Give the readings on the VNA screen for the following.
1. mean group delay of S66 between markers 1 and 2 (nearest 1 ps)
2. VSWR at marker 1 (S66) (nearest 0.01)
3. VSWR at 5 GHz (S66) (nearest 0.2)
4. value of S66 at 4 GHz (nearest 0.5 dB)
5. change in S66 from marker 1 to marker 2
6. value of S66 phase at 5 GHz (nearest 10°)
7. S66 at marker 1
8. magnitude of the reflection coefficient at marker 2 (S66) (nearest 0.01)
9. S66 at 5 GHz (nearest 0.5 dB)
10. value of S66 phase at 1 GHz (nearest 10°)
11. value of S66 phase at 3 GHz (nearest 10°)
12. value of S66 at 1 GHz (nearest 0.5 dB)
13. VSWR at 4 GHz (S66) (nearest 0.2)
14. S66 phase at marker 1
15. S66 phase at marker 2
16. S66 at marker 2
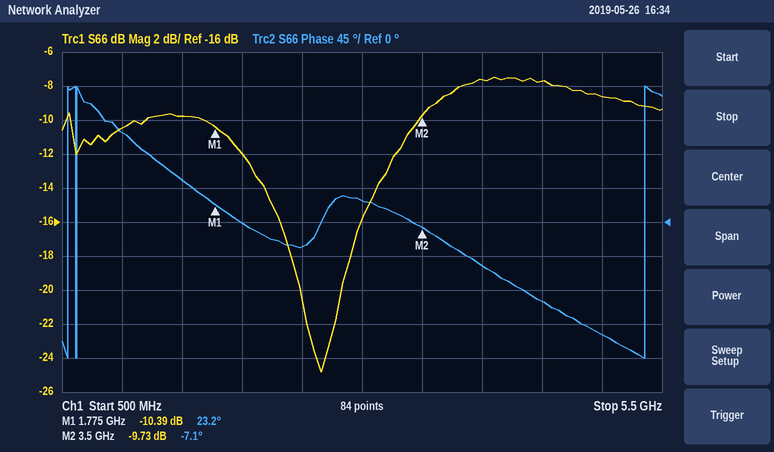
49 ps
1.87
2.2
-7.5 dB
0.66 dB
-150°
-10.39 dB
0.33
-8.5 dB
120°
30°
-10.5 dB
2.4
23.2°
-7.1°
-9.73 dB
